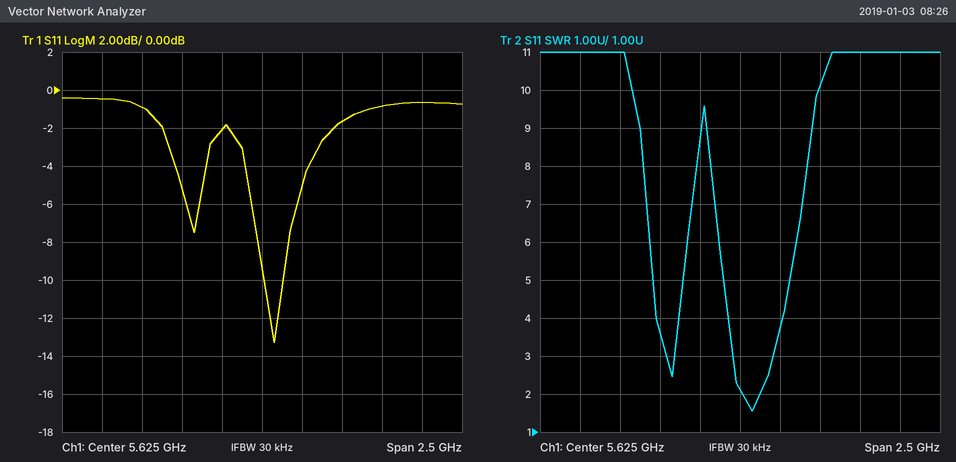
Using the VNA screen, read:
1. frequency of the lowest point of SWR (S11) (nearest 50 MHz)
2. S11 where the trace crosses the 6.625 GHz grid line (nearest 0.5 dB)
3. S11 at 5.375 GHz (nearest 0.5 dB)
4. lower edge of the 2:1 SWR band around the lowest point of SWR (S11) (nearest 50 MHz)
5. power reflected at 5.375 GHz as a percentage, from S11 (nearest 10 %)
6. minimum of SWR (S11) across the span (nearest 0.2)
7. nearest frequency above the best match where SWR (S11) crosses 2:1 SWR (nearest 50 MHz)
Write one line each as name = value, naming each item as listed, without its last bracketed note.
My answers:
frequency of the lowest point of SWR (S11) = 5.70 GHz
S11 where the trace crosses the 6.625 GHz grid line = -0.5 dB
S11 at 5.375 GHz = -2.0 dB
lower edge of the 2:1 SWR band around the lowest point of SWR (S11) = 5.65 GHz
power reflected at 5.375 GHz as a percentage, from S11 = 60 %
minimum of SWR (S11) across the span = 1.6
nearest frequency above the best match where SWR (S11) crosses 2:1 SWR = 5.75 GHz
